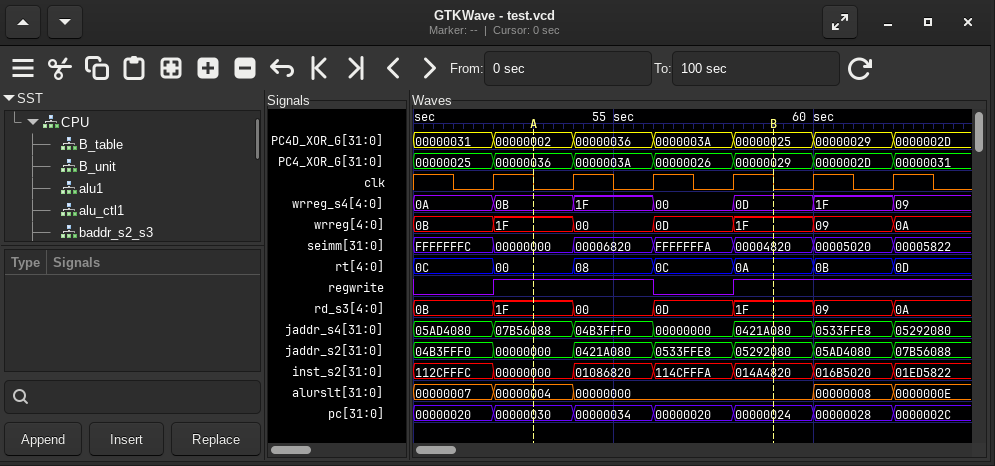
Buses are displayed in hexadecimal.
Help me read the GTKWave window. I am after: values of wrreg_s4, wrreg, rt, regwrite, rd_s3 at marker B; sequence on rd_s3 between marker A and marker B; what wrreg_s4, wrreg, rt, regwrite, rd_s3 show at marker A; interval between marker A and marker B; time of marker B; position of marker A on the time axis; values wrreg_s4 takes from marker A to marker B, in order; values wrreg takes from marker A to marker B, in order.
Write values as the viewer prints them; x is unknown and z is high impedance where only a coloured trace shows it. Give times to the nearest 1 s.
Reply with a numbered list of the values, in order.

1. wrreg_s4=0D, wrreg=1F, rt=0A, regwrite=1, rd_s3=1F
2. 1F, 00, 0D, 1F
3. wrreg_s4=0B, wrreg=1F, rt=00, regwrite=1, rd_s3=1F
4. 6 s
5. 59 s
6. 53 s
7. 0B, 1F, 00, 0D
8. 1F, 00, 0D, 1F
